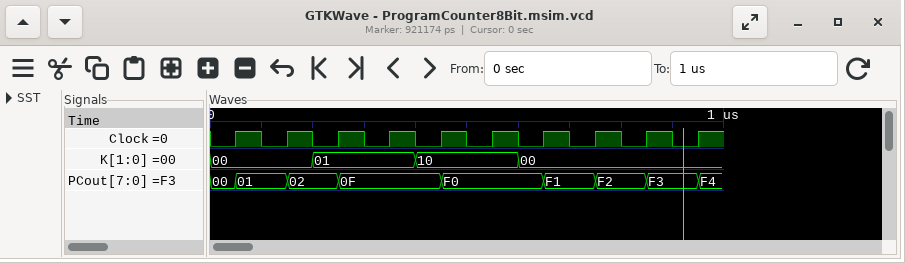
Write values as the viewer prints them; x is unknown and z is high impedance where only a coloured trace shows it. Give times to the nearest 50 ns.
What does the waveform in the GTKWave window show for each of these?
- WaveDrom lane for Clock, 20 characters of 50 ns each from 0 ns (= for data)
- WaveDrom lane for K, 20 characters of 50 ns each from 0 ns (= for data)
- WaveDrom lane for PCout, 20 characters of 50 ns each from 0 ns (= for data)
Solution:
{name: 'Clock', wave: '01010101010101010101'}
{name: 'K', wave: '=...=...=...=.......', data: '00 01 10 00'}
{name: 'PCout', wave: '==.=.=...=...=.=.=.=', data: '00 01 02 0F F0 F1 F2 F3 F4'}
